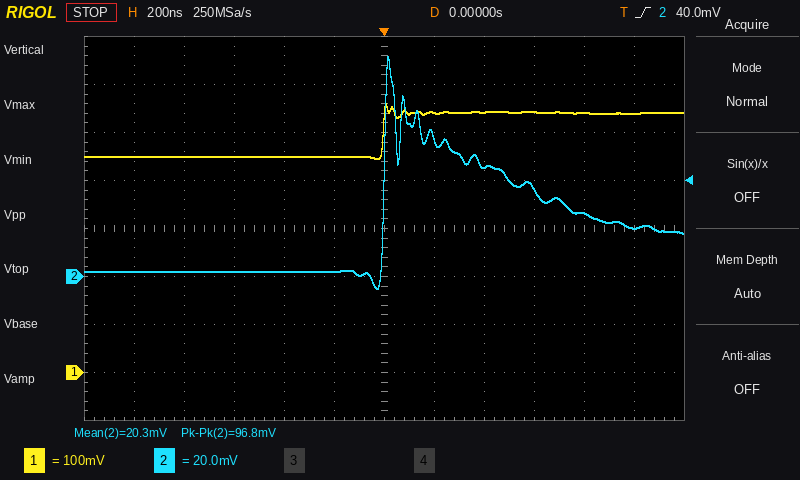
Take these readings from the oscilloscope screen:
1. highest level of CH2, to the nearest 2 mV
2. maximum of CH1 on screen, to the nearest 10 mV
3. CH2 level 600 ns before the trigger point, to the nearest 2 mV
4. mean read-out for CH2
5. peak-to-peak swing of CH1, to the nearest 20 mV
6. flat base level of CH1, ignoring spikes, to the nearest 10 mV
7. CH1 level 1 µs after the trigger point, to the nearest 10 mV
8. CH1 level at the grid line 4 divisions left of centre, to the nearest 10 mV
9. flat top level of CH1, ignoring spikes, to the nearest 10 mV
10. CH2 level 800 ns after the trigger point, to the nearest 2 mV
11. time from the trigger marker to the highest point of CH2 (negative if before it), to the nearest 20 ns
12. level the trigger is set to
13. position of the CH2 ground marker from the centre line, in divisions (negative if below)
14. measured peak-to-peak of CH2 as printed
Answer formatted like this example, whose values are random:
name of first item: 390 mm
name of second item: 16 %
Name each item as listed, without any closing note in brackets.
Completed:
highest level of CH2, to the nearest 2 mV: 92 mV
maximum of CH1 on screen, to the nearest 10 mV: 560 mV
CH2 level 600 ns before the trigger point, to the nearest 2 mV: 2 mV
mean read-out for CH2: 20.3 mV
peak-to-peak swing of CH1, to the nearest 20 mV: 120 mV
flat base level of CH1, ignoring spikes, to the nearest 10 mV: 450 mV
CH1 level 1 µs after the trigger point, to the nearest 10 mV: 540 mV
CH1 level at the grid line 4 divisions left of centre, to the nearest 10 mV: 450 mV
flat top level of CH1, ignoring spikes, to the nearest 10 mV: 540 mV
CH2 level 800 ns after the trigger point, to the nearest 2 mV: 26 mV
time from the trigger marker to the highest point of CH2 (negative if before it), to the nearest 20 ns: +20 ns
level the trigger is set to: 40.0 mV
position of the CH2 ground marker from the centre line, in divisions: -1.0 div
measured peak-to-peak of CH2 as printed: 96.8 mV
